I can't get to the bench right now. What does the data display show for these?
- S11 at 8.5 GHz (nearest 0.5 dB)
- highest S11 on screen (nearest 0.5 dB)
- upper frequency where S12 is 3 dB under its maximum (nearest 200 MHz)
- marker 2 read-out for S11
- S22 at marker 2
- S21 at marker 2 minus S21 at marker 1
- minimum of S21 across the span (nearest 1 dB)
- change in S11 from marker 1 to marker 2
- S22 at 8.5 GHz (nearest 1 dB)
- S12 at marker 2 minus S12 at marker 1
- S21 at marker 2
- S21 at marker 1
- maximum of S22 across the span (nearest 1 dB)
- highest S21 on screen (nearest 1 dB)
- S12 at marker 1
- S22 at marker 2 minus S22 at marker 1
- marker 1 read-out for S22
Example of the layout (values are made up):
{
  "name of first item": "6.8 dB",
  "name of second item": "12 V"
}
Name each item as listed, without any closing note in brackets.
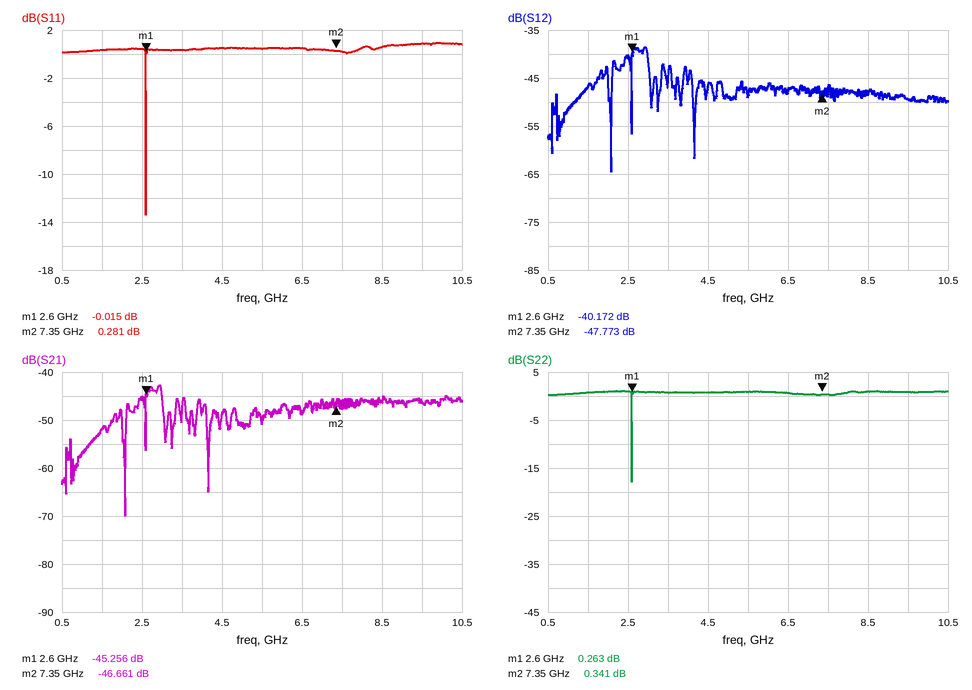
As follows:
{
  "S11 at 8.5 GHz": "0.5 dB",
  "highest S11 on screen": "1.0 dB",
  "upper frequency where S12 is 3 dB under its maximum": "3.0 GHz",
  "marker 2 read-out for S11": "0.281 dB",
  "S22 at marker 2": "0.341 dB",
  "S21 at marker 2 minus S21 at marker 1": "-1.405 dB",
  "minimum of S21 across the span": "-70 dB",
  "change in S11 from marker 1 to marker 2": "0.296 dB",
  "S22 at 8.5 GHz": "1 dB",
  "S12 at marker 2 minus S12 at marker 1": "-7.601 dB",
  "S21 at marker 2": "-46.661 dB",
  "S21 at marker 1": "-45.256 dB",
  "maximum of S22 across the span": "1 dB",
  "highest S21 on screen": "-43 dB",
  "S12 at marker 1": "-40.172 dB",
  "S22 at marker 2 minus S22 at marker 1": "0.078 dB",
  "marker 1 read-out for S22": "0.263 dB"
}
